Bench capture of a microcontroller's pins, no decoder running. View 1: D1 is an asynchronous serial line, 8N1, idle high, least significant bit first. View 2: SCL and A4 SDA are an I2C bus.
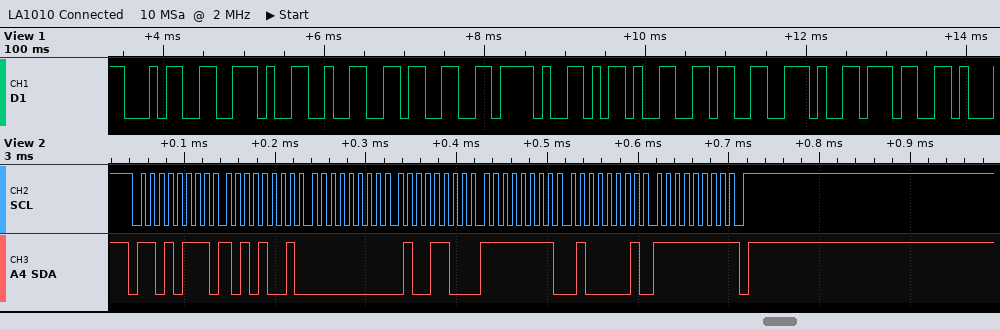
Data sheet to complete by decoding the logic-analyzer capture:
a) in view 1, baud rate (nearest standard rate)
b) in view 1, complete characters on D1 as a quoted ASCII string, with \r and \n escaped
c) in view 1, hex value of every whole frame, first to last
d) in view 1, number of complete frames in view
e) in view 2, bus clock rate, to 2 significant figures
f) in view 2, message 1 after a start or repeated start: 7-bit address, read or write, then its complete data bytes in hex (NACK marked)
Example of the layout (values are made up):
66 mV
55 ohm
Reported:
9600 baud
"4.23/-6.7"
0x34 0x2E 0x32 0x33 0x2F 0x2D 0x36 0x2E 0x37
9
100 kHz
0x6B read: A9 00 4C FF 41 FF NACK
